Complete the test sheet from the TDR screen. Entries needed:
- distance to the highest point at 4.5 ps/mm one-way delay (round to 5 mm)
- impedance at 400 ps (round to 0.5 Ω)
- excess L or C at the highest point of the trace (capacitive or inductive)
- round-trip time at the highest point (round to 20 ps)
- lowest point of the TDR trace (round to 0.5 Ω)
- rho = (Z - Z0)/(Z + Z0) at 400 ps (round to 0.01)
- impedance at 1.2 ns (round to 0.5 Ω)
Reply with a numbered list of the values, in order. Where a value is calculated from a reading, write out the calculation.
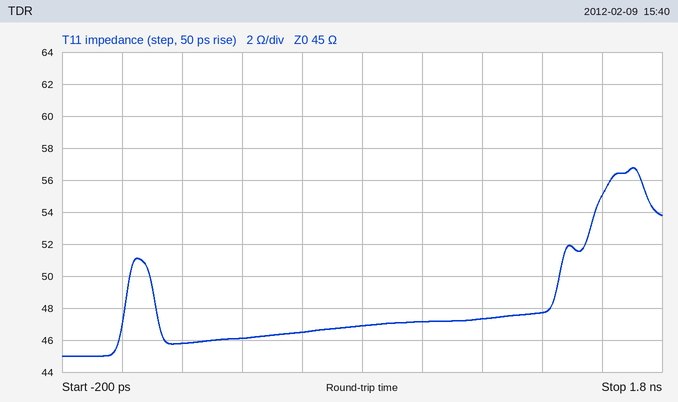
1. 1.70 ns / 2 / 4.5 ps/mm ≈ 189 mm, so 190 mm to the nearest 5 mm
2. 46.0 Ω
3. inductive
4. 1.70 ns
5. 45.0 Ω
6. (46 − 45)/(46 + 45) ≈ +0.01
7. 47.5 Ω
